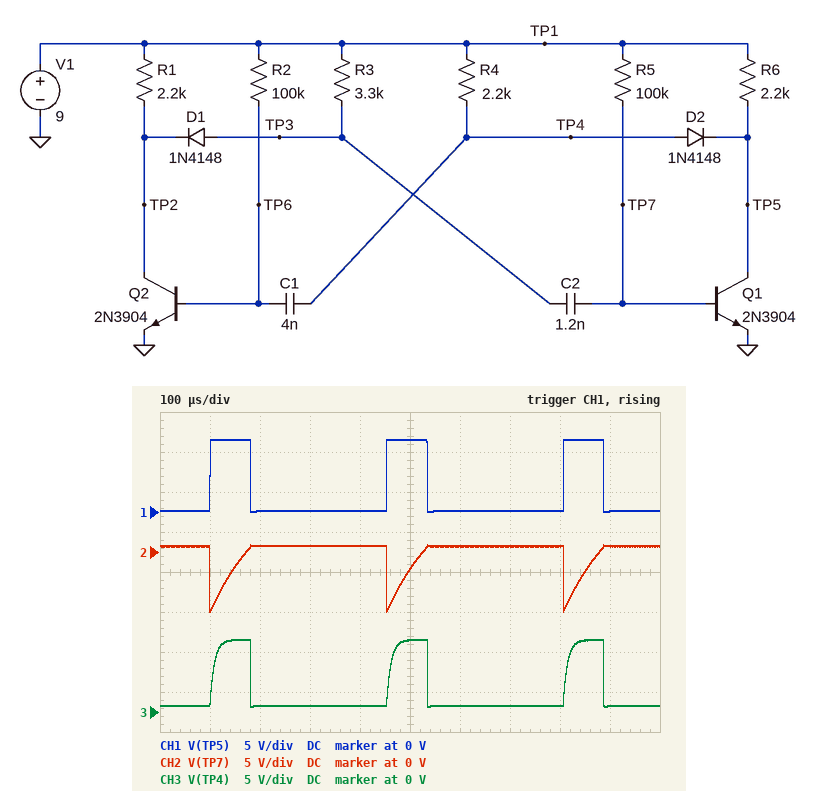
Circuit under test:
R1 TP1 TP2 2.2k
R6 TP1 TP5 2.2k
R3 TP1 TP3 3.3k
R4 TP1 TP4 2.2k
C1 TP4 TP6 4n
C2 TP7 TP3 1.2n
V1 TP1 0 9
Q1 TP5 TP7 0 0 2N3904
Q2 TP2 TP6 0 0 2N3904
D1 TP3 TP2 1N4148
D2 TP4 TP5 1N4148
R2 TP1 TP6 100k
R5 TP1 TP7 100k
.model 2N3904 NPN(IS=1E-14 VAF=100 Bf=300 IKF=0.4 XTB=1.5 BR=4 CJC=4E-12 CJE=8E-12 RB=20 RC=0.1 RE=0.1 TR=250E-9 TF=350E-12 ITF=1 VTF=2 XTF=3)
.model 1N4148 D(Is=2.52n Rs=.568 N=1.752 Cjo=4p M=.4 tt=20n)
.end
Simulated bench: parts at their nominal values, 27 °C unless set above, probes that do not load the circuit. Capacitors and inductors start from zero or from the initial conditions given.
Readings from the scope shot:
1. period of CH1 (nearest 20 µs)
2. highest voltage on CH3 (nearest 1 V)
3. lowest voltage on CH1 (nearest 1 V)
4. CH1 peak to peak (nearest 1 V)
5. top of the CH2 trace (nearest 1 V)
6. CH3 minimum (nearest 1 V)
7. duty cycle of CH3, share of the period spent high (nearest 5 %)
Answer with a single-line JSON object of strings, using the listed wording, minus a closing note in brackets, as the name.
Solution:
{"period of CH1": "360 µs", "highest voltage on CH3": "9 V", "lowest voltage on CH1": "0 V", "CH1 peak to peak": "9 V", "top of the CH2 trace": "1 V", "CH3 minimum": "1 V", "duty cycle of CH3, share of the period spent high": "20 %"}
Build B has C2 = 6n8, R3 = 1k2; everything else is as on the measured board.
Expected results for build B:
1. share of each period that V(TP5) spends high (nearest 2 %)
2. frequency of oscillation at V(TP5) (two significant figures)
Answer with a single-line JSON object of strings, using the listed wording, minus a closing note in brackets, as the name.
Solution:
{"share of each period that V(TP5) spends high": "62 %", "frequency of oscillation at V(TP5)": "1.4 kHz"}
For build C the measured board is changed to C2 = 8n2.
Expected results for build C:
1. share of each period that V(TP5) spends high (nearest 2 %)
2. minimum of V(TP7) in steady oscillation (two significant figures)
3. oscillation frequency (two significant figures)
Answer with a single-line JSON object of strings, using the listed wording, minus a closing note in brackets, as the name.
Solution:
{"share of each period that V(TP5) spends high": "68 %", "minimum of V(TP7) in steady oscillation": "-7.6 V", "oscillation frequency": "1.2 kHz"}
